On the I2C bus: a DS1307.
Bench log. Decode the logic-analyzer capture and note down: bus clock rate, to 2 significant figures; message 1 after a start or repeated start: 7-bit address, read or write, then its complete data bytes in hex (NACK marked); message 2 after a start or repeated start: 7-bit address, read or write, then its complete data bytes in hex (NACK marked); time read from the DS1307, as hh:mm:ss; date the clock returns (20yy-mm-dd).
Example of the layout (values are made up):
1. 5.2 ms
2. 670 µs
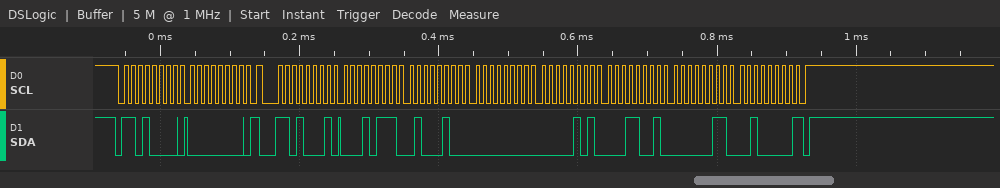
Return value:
1. 100 kHz
2. 0x68 write: 00
3. 0x68 read: 17 44 00 05 19 03 20 NACK
4. 00:44:17
5. 2020-03-19
